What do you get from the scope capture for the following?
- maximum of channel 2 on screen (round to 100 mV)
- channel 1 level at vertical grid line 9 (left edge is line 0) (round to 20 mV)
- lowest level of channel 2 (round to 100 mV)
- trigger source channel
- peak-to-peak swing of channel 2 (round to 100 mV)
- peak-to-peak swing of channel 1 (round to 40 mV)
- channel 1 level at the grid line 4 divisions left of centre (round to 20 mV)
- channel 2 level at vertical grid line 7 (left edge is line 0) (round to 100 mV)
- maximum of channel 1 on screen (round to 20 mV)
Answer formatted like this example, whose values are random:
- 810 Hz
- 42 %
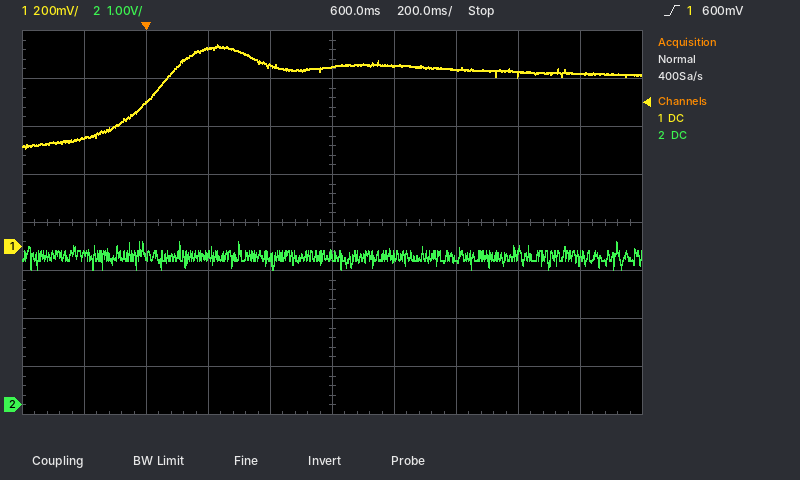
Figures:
- 3.4 V
- 720 mV
- 2.8 V
- channel 1
- 600 mV
- 440 mV
- 460 mV
- 3.0 V
- 840 mV
